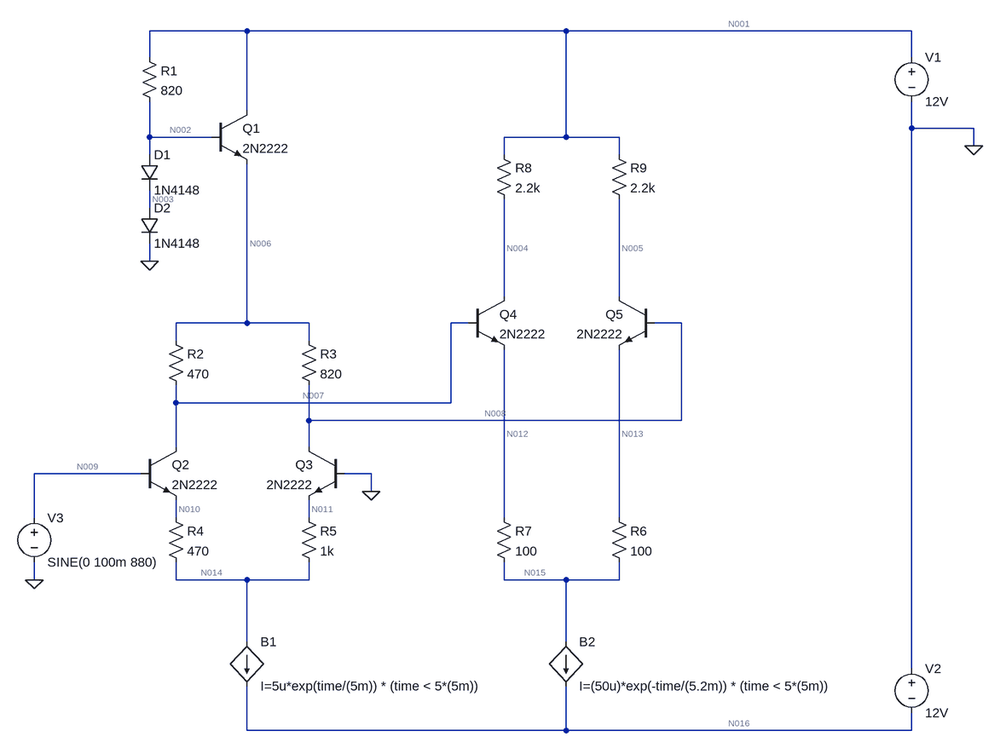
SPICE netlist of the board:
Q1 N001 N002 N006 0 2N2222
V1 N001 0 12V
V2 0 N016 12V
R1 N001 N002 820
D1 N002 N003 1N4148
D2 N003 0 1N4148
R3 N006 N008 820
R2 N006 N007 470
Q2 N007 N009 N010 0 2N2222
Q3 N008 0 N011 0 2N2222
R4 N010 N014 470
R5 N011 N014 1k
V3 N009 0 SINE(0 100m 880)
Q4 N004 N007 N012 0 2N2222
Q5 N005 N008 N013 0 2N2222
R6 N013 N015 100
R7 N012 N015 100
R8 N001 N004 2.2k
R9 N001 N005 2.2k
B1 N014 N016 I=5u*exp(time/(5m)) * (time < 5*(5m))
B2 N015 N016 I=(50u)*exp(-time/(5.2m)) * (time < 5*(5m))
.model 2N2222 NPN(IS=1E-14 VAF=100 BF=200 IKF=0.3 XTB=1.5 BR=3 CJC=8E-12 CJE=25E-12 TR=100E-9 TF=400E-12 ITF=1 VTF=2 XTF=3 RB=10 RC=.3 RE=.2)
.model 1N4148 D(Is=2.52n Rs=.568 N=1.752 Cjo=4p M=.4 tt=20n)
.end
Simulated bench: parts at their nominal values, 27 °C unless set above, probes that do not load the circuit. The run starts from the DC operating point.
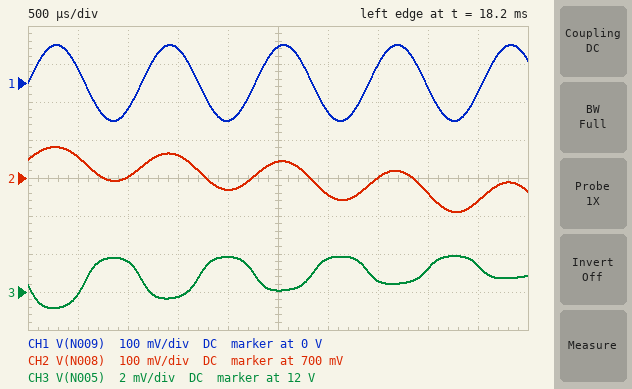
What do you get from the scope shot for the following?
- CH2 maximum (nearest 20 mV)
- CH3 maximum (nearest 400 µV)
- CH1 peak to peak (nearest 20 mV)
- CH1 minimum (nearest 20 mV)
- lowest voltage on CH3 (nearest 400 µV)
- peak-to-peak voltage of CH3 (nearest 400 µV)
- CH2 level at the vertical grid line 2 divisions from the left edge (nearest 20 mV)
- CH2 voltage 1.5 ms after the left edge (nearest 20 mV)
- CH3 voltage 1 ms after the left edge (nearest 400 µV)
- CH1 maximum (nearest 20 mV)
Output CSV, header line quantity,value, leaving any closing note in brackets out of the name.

quantity,value
CH2 maximum,780 mV
CH3 maximum,12.0000 V
CH1 peak to peak,200 mV
CH1 minimum,-100 mV
lowest voltage on CH3,11.9972 V
peak-to-peak voltage of CH3,2.8 mV
CH2 level at the vertical grid line 2 divisions from the left edge,700 mV
CH2 voltage 1.5 ms after the left edge,760 mV
CH3 voltage 1 ms after the left edge,11.9996 V
CH1 maximum,100 mV
